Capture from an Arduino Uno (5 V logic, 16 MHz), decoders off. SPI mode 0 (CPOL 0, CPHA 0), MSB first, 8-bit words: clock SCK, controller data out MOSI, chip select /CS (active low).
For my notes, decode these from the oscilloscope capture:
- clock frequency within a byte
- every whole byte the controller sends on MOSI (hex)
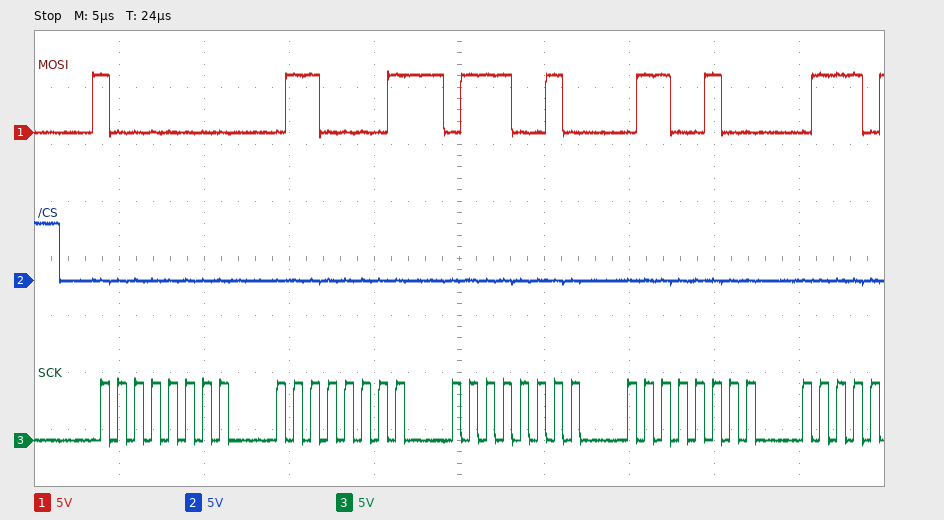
1 MHz
80 61 72 64
